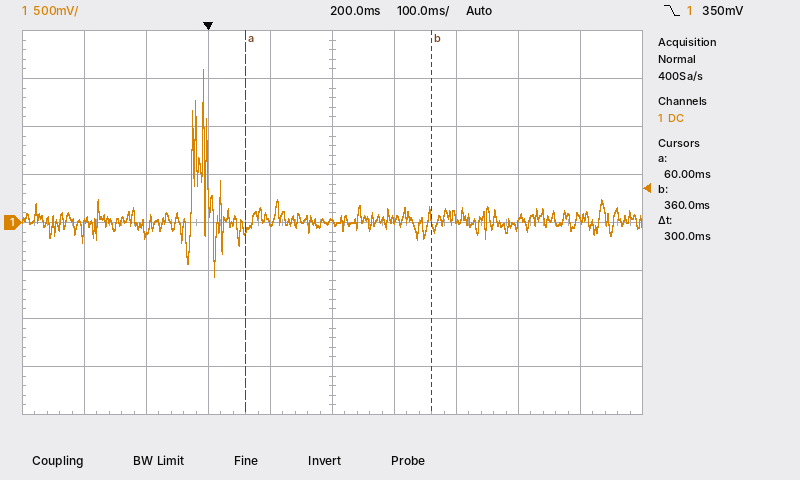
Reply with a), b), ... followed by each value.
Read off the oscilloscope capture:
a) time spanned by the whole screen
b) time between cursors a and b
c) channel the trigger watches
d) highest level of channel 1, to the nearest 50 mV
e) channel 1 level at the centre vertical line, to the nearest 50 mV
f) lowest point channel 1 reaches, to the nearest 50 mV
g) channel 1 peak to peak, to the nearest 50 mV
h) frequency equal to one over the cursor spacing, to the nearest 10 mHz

a) 1 s
b) 300 ms
c) channel 1
d) 1.60 V
e) 0 mV
f) -550 mV
g) 2.15 V
h) 3.33 Hz
